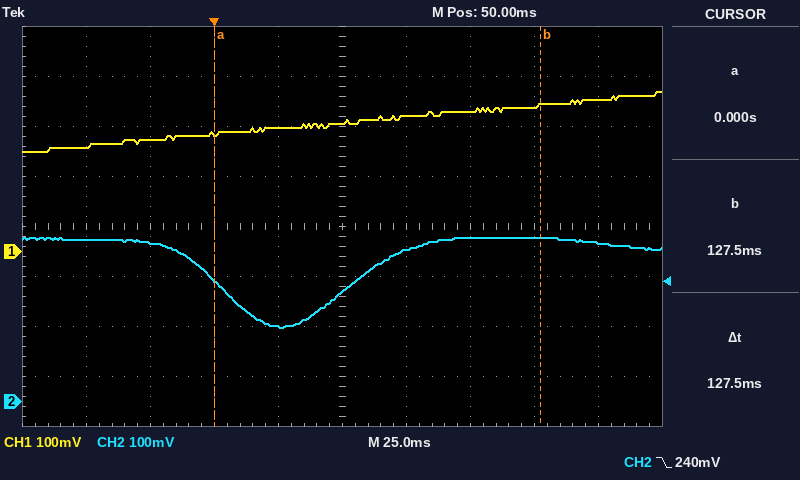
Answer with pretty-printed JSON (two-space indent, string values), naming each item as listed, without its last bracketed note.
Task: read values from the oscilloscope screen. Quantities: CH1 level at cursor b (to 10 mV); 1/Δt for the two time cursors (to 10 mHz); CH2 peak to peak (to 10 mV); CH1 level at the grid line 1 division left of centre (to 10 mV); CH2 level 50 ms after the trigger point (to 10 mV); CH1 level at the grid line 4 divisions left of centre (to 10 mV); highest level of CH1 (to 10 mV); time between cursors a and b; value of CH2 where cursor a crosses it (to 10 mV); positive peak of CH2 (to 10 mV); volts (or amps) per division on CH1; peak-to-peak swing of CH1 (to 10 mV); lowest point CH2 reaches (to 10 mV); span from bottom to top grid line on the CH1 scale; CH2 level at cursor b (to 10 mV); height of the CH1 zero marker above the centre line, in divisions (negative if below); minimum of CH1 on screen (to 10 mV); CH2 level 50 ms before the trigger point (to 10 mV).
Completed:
{
  "CH1 level at cursor b": "290 mV",
  "1/Δt for the two time cursors": "7.84 Hz",
  "CH2 peak to peak": "180 mV",
  "CH1 level at the grid line 1 division left of centre": "250 mV",
  "CH2 level 50 ms after the trigger point": "220 mV",
  "CH1 level at the grid line 4 divisions left of centre": "210 mV",
  "highest level of CH1": "320 mV",
  "time between cursors a and b": "127.5 ms",
  "value of CH2 where cursor a crosses it": "240 mV",
  "positive peak of CH2": "330 mV",
  "volts (or amps) per division on CH1": "100 mV",
  "peak-to-peak swing of CH1": "120 mV",
  "lowest point CH2 reaches": "150 mV",
  "span from bottom to top grid line on the CH1 scale": "800 mV",
  "CH2 level at cursor b": "330 mV",
  "height of the CH1 zero marker above the centre line, in divisions": "-0.5 div",
  "minimum of CH1 on screen": "200 mV",
  "CH2 level 50 ms before the trigger point": "320 mV"
}
